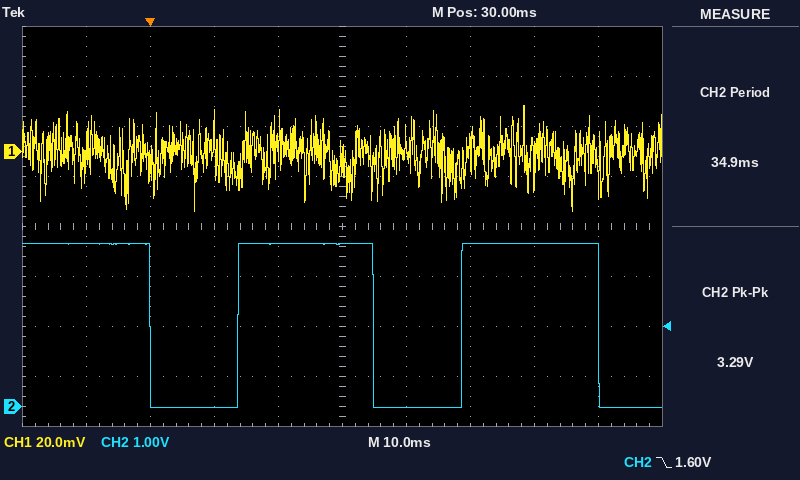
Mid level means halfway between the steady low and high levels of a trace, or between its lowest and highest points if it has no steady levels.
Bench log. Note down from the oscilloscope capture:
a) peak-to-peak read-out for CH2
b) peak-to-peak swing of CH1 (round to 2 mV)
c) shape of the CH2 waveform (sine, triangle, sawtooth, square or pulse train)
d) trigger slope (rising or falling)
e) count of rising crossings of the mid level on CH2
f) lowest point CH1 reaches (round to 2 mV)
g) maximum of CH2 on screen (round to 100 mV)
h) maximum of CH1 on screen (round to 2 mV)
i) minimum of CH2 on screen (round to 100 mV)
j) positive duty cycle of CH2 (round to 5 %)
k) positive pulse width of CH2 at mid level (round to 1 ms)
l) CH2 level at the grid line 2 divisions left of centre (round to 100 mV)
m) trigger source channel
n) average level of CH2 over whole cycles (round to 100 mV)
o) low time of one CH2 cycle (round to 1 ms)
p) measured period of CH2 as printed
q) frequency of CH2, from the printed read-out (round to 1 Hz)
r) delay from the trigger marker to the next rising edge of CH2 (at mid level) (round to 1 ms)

3.29 V
42 mV
pulse train
falling
2
-24 mV
3.3 V
18 mV
0.0 V
60 %
21 ms
0.0 V
CH2
2.0 V
14 ms
34.9 ms
29 Hz
14 ms
